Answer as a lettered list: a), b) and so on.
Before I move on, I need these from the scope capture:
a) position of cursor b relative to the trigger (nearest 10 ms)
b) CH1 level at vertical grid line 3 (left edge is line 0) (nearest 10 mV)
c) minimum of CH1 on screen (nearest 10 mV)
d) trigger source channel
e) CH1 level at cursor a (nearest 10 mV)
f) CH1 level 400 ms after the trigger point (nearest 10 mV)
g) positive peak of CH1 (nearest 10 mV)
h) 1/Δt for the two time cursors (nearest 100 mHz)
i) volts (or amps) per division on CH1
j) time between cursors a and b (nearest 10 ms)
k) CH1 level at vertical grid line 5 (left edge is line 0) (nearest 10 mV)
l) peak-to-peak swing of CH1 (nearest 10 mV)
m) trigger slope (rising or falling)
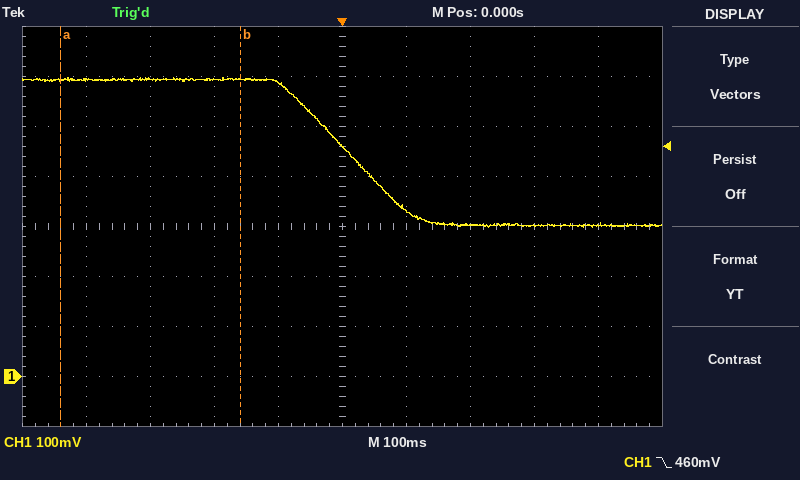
a) -160 ms
b) 590 mV
c) 300 mV
d) CH1
e) 590 mV
f) 300 mV
g) 600 mV
h) 3.6 Hz
i) 100 mV
j) 280 ms
k) 460 mV
l) 300 mV
m) falling
